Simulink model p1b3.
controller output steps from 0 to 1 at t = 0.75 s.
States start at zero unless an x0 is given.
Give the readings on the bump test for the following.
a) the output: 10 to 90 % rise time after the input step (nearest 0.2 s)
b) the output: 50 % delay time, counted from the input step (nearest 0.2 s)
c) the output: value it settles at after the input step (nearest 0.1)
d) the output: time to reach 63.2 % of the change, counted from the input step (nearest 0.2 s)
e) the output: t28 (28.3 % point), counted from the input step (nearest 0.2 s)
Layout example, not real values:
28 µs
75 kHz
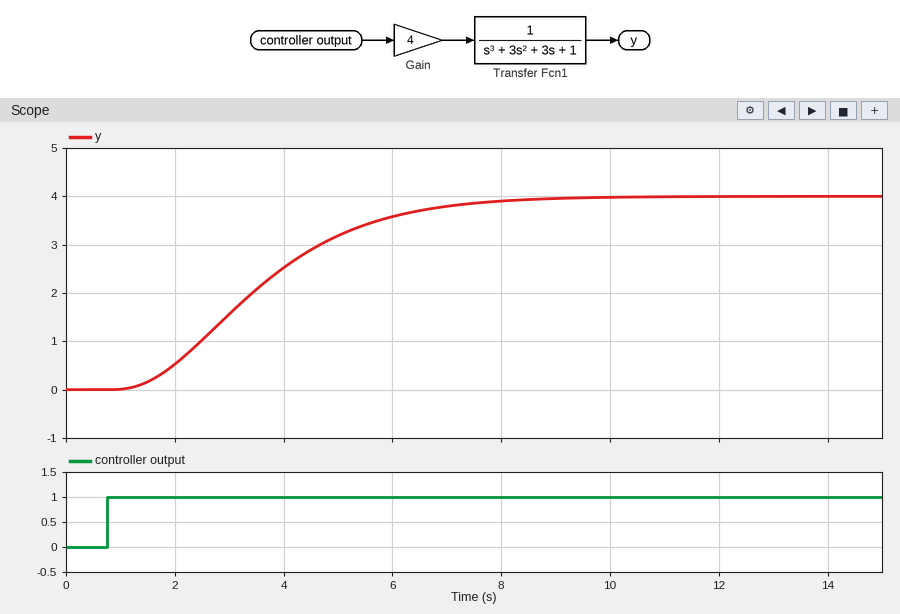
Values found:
4.2 s
2.6 s
4.0
3.2 s
1.8 s
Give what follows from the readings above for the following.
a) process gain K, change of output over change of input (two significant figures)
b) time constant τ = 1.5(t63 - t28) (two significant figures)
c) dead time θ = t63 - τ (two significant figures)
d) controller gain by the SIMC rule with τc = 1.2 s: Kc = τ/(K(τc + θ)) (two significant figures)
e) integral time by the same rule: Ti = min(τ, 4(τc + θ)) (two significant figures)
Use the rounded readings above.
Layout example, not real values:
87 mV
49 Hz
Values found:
4.0
2.1 s
1.1 s
0.23
2.1 s
